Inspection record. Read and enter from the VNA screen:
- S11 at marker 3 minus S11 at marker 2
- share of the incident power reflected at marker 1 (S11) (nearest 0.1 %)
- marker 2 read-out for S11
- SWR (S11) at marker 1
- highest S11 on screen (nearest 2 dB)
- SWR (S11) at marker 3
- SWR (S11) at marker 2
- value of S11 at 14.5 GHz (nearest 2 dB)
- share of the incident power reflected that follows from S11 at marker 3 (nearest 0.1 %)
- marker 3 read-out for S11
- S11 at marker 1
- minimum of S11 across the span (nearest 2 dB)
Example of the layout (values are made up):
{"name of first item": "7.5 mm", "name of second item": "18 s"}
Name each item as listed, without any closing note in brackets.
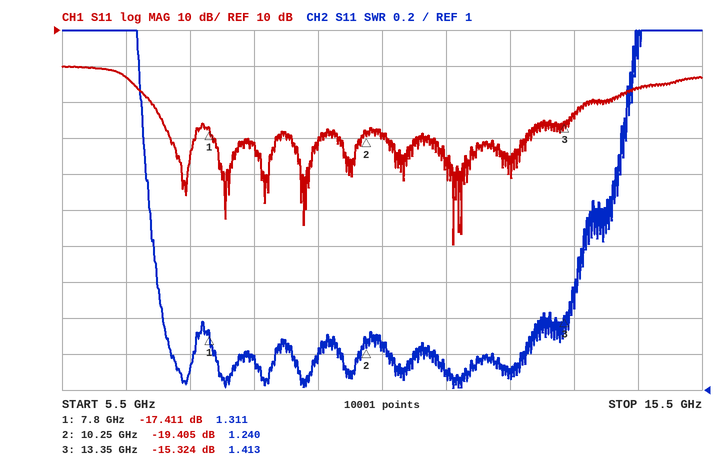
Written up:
{"S11 at marker 3 minus S11 at marker 2": "4.081 dB", "share of the incident power reflected at marker 1 (S11)": "1.8 %", "marker 2 read-out for S11": "-19.405 dB", "SWR (S11) at marker 1": "1.311", "highest S11 on screen": "0 dB", "SWR (S11) at marker 3": "1.413", "SWR (S11) at marker 2": "1.240", "value of S11 at 14.5 GHz": "-6 dB", "share of the incident power reflected that follows from S11 at marker 3": "2.9 %", "marker 3 read-out for S11": "-15.324 dB", "S11 at marker 1": "-17.411 dB", "minimum of S11 across the span": "-50 dB"}
